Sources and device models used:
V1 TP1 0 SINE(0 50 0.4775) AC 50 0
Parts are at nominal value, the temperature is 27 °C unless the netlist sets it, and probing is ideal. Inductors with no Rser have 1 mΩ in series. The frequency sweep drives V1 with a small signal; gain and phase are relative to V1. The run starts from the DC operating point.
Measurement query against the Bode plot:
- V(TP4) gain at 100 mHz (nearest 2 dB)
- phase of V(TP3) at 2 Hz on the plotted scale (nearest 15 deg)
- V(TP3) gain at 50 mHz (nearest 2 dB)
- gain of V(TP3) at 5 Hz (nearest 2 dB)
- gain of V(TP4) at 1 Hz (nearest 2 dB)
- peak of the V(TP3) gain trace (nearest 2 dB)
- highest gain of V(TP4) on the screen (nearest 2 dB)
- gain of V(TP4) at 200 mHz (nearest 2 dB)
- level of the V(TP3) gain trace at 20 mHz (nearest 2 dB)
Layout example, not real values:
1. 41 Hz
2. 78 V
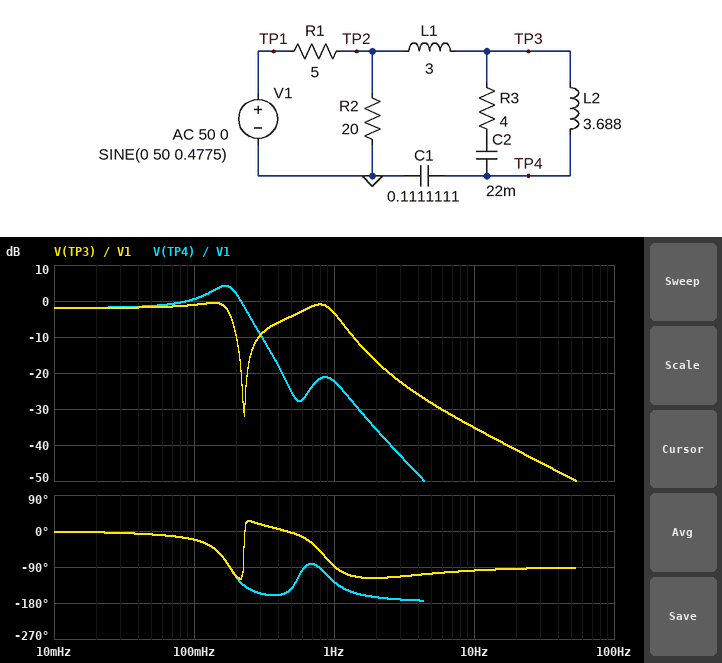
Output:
1. 0 dB
2. -120 deg
3. -2 dB
4. -28 dB
5. -22 dB
6. 0 dB
7. 4 dB
8. 2 dB
9. -2 dB
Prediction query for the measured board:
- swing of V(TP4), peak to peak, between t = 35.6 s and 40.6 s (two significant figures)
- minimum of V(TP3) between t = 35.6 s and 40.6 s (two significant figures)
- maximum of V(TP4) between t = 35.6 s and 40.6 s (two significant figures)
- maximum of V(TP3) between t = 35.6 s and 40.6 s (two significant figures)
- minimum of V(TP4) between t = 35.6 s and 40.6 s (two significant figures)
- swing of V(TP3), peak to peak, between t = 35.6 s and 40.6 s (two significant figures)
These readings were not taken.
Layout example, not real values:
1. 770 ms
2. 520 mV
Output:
1. 6.4 V
2. -30 V
3. 3.2 V
4. 30 V
5. -3.2 V
6. 59 V
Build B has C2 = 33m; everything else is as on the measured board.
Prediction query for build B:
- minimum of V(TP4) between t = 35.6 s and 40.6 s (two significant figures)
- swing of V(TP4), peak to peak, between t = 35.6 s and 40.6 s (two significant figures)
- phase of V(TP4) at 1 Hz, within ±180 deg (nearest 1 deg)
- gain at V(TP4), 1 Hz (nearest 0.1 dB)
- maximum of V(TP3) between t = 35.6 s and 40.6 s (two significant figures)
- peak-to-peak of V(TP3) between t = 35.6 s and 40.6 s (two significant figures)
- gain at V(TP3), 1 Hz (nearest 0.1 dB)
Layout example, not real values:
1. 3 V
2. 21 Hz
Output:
1. -3.5 V
2. 7.0 V
3. -141 deg
4. -23.0 dB
5. 34 V
6. 67 V
7. -7.3 dB
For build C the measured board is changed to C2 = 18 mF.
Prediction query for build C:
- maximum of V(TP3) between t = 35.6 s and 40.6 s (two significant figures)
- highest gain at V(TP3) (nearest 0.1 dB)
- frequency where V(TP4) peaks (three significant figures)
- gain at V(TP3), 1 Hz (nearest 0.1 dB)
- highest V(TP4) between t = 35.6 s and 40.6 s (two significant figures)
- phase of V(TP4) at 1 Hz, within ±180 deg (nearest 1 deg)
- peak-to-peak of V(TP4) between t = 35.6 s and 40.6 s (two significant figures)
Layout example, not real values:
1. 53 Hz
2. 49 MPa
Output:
1. 28 V
2. -0.3 dB
3. 169 mHz
4. -1.2 dB
5. 3.8 V
6. -113 deg
7. 7.6 V
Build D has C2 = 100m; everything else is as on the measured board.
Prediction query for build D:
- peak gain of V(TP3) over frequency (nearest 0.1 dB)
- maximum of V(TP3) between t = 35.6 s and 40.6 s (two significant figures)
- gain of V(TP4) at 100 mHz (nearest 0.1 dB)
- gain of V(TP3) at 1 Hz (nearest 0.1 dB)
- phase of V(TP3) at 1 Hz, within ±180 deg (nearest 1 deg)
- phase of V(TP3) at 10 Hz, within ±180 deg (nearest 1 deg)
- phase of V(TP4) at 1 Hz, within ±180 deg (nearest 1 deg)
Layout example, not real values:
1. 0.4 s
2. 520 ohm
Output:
1. -0.9 dB
2. 27 V
3. 0.7 dB
4. -13.3 dB
5. -90 deg
6. -91 deg
7. -153 deg
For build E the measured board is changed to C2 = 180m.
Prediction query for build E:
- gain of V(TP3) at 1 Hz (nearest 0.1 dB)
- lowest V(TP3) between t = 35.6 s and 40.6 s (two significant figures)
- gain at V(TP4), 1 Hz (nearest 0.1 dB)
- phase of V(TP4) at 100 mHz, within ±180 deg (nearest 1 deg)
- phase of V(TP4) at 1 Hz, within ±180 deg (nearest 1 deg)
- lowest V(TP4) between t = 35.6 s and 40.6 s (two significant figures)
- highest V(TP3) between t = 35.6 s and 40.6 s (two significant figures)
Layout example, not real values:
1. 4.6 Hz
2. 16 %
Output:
1. -14.5 dB
2. -22 V
3. -24.4 dB
4. -25 deg
5. -155 deg
6. -11 V
7. 22 V
